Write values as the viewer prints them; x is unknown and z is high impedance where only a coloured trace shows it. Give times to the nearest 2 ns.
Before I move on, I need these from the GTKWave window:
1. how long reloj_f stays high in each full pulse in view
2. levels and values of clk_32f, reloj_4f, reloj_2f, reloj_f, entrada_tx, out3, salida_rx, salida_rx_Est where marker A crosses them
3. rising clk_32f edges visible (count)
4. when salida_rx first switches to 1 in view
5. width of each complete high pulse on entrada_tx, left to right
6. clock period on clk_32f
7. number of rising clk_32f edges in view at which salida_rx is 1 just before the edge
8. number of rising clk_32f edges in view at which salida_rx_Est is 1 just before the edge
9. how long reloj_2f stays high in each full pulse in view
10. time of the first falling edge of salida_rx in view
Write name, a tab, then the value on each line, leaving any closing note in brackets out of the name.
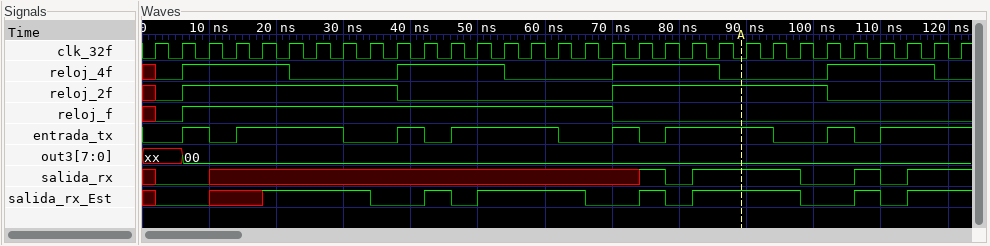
how long reloj_f stays high in each full pulse in view	64 ns
levels and values of clk_32f, reloj_4f, reloj_2f, reloj_f, entrada_tx, out3, salida_rx, salida_rx_Est where marker A crosses them	clk_32f=0, reloj_4f=0, reloj_2f=1, reloj_f=0, entrada_tx=1, out3=00, salida_rx=1, salida_rx_Est=1
rising clk_32f edges visible	31
when salida_rx first switches to 1 in view	74 ns
width of each complete high pulse on entrada_tx, left to right	4 ns, 16 ns, 4 ns, 16 ns, 4 ns, 16 ns, 4 ns
clock period on clk_32f	4 ns
number of rising clk_32f edges in view at which salida_rx is 1 just before the edge	8
number of rising clk_32f edges in view at which salida_rx_Est is 1 just before the edge	17
how long reloj_2f stays high in each full pulse in view	32 ns, 32 ns
time of the first falling edge of salida_rx in view	78 ns
